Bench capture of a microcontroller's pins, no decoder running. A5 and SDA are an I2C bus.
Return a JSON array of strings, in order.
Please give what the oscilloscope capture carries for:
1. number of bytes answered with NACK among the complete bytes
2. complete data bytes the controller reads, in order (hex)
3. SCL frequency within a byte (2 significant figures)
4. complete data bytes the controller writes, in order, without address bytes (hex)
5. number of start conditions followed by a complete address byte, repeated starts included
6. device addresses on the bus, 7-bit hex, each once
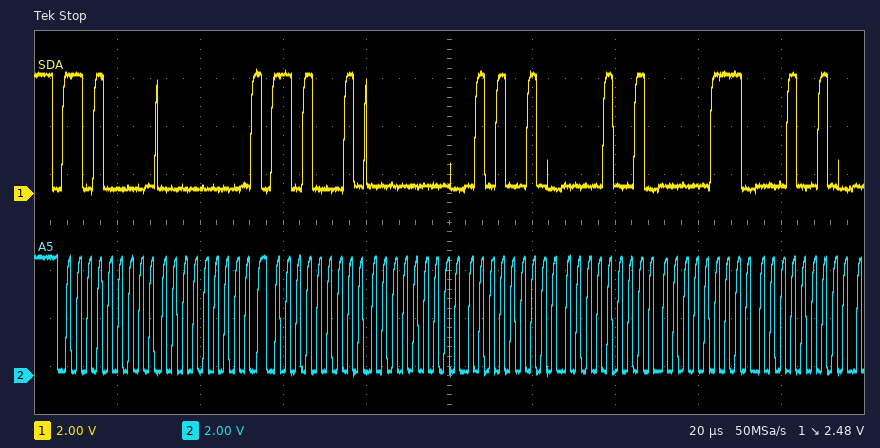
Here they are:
["0", "00 52 09 07 12", "400 kHz", "00", "2", "0x68"]
